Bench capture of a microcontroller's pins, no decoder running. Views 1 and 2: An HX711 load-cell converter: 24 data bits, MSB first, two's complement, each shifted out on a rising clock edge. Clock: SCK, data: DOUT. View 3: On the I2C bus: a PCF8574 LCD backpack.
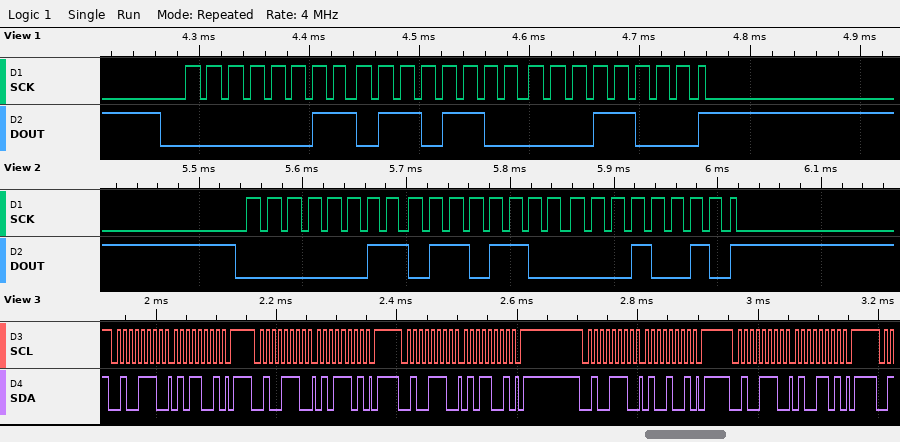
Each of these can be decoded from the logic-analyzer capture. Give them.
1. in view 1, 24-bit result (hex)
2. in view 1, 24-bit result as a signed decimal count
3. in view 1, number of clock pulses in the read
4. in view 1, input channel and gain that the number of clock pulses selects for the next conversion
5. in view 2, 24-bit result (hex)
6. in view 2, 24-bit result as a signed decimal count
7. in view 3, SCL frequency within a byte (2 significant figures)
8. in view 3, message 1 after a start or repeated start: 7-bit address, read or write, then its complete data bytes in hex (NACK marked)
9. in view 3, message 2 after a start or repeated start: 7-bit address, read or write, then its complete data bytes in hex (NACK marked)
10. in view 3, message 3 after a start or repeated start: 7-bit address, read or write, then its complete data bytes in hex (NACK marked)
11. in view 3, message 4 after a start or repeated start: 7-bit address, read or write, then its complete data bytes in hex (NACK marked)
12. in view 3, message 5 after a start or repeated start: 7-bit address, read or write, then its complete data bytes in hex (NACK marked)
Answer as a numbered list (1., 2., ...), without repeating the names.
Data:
1. 0x036C18
2. 224280
3. 25
4. channel A, gain 128
5. 0x036C12
6. 224274
7. 100 kHz
8. 0x27 write: 59
9. 0x27 write: 5D
10. 0x27 write: 59
11. 0x27 write: 49
12. 0x27 write: 4D
